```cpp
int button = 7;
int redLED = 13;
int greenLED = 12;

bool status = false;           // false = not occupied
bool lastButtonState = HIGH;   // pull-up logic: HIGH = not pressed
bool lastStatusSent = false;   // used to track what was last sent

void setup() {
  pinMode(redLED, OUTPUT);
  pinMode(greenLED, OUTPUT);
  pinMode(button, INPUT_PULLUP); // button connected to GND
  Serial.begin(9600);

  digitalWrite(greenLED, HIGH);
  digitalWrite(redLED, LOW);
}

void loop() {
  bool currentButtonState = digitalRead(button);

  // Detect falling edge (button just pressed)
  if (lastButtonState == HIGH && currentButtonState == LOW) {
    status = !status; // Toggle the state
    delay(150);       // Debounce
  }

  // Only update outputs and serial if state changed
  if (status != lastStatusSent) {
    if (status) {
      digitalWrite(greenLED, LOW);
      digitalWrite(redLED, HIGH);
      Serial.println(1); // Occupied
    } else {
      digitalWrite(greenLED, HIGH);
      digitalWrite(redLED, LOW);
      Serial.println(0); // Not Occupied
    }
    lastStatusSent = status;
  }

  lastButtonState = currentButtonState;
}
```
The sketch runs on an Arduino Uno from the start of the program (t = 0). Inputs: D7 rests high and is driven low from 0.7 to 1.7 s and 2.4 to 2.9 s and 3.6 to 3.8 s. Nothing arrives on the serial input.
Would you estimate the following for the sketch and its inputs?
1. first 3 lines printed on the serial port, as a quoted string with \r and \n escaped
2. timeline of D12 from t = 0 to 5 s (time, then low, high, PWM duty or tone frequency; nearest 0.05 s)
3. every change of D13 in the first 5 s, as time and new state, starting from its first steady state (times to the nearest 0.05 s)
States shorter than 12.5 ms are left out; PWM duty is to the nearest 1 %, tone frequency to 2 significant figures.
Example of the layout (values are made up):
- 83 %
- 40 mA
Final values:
- "1\r\n0\r\n1\r\n"
- 0 s high; 0.85 s low; 2.55 s high; 3.75 s low
- 0 s low; 0.85 s high; 2.55 s low; 3.75 s high
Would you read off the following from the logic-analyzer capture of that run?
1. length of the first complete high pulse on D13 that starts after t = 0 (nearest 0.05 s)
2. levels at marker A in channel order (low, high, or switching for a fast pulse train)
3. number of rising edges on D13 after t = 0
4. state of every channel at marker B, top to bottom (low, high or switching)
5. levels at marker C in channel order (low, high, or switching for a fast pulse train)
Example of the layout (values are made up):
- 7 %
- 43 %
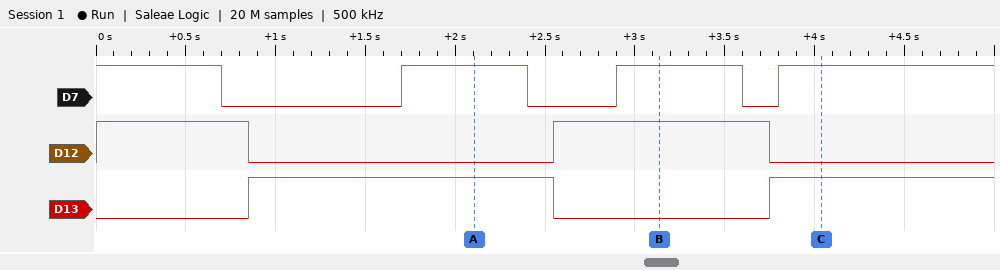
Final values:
- 1.70 s
- D7 high, D12 low, D13 high
- 2
- D7 high, D12 high, D13 low
- D7 high, D12 low, D13 high
